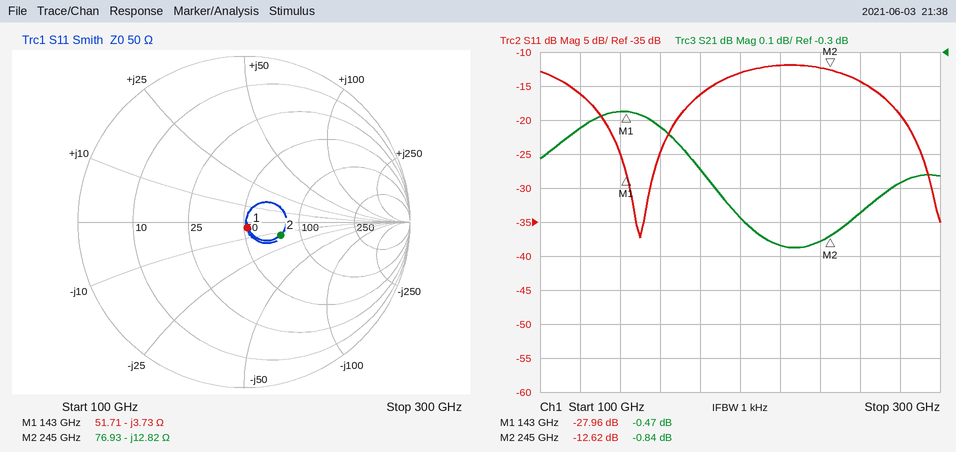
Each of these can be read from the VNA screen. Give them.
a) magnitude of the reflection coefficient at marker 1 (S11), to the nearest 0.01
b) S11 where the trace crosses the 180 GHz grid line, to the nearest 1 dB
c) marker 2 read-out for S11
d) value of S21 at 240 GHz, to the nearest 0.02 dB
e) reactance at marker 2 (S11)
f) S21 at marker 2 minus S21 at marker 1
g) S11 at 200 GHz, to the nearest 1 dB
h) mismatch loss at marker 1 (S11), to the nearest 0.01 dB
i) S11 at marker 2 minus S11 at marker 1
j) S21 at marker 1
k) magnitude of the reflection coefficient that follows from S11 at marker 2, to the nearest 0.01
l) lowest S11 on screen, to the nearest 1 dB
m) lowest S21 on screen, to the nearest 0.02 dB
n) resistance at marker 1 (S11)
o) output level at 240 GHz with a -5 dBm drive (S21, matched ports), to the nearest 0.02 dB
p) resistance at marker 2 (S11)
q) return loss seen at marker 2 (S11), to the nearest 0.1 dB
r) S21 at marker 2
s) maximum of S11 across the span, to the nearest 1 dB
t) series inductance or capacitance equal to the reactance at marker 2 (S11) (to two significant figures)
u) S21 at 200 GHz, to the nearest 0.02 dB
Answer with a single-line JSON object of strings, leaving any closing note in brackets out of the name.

{"magnitude of the reflection coefficient at marker 1 (S11), to the nearest 0.01": "0.04", "S11 where the trace crosses the 180 GHz grid line, to the nearest 1 dB": "-16 dB", "marker 2 read-out for S11": "-12.62 dB", "value of S21 at 240 GHz, to the nearest 0.02 dB": "-0.86 dB", "reactance at marker 2": "-12.82 Ω", "S21 at marker 2 minus S21 at marker 1": "-0.37 dB", "S11 at 200 GHz, to the nearest 1 dB": "-13 dB", "mismatch loss at marker 1 (S11), to the nearest 0.01 dB": "0.01 dB", "S11 at marker 2 minus S11 at marker 1": "15.34 dB", "S21 at marker 1": "-0.47 dB", "magnitude of the reflection coefficient that follows from S11 at marker 2, to the nearest 0.01": "0.23", "lowest S11 on screen, to the nearest 1 dB": "-37 dB", "lowest S21 on screen, to the nearest 0.02 dB": "-0.88 dB", "resistance at marker 1": "51.71 Ω", "output level at 240 GHz with a -5 dBm drive (S21, matched ports), to the nearest 0.02 dB": "-5.86 dBm", "resistance at marker 2": "76.93 Ω", "return loss seen at marker 2 (S11), to the nearest 0.1 dB": "12.6 dB", "S21 at marker 2": "-0.84 dB", "maximum of S11 across the span, to the nearest 1 dB": "-12 dB", "series inductance or capacitance equal to the reactance at marker 2 (S11)": "51 fF", "S21 at 200 GHz, to the nearest 0.02 dB": "-0.78 dB"}
